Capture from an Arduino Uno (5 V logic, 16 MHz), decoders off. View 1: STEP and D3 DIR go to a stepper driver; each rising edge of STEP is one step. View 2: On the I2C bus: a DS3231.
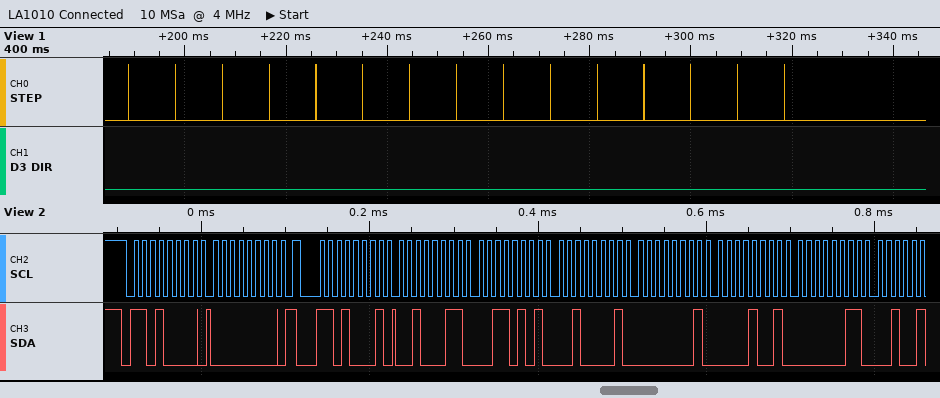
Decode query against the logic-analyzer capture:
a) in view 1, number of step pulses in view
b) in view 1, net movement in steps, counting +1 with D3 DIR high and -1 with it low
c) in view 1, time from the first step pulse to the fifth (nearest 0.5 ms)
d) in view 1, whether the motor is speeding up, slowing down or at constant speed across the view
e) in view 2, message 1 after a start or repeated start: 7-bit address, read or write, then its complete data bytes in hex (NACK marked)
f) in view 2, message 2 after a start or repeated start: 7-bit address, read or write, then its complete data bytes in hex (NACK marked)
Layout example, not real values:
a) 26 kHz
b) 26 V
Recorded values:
a) 15
b) -15
c) 37.0 ms
d) constant speed
e) 0x68 write: 00
f) 0x68 read: 23 35 21 01 09 03
